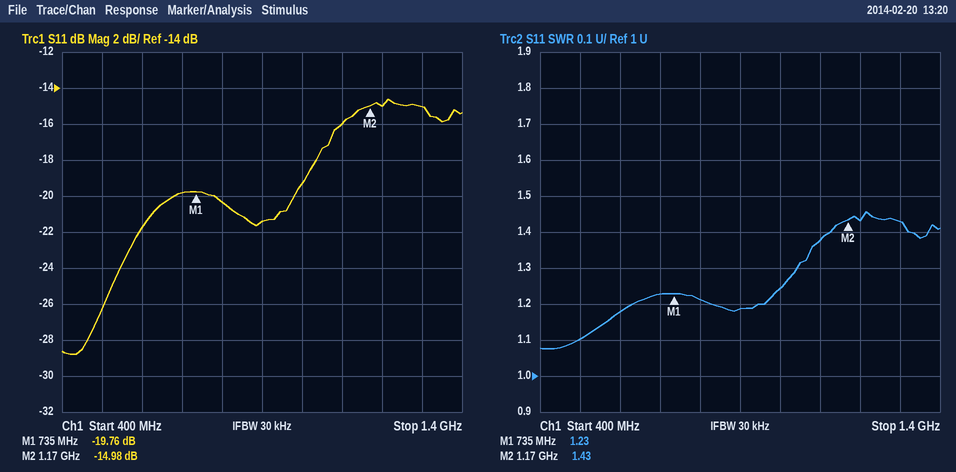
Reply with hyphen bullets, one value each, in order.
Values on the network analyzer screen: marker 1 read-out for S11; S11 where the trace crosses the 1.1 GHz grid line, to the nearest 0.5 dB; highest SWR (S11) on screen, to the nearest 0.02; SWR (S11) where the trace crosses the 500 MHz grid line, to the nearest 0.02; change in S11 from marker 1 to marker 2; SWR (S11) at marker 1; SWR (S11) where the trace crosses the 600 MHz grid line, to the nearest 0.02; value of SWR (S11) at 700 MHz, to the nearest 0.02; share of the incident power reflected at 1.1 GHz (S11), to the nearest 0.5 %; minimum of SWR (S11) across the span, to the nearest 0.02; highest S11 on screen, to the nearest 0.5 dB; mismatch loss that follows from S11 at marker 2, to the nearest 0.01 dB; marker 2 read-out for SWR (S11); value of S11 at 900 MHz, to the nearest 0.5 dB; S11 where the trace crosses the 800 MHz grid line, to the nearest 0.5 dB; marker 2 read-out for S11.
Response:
- -19.76 dB
- -16.0 dB
- 1.46
- 1.10
- 4.78 dB
- 1.23
- 1.18
- 1.22
- 2.5 %
- 1.08
- -14.5 dB
- 0.14 dB
- 1.43
- -21.5 dB
- -20.5 dB
- -14.98 dB
